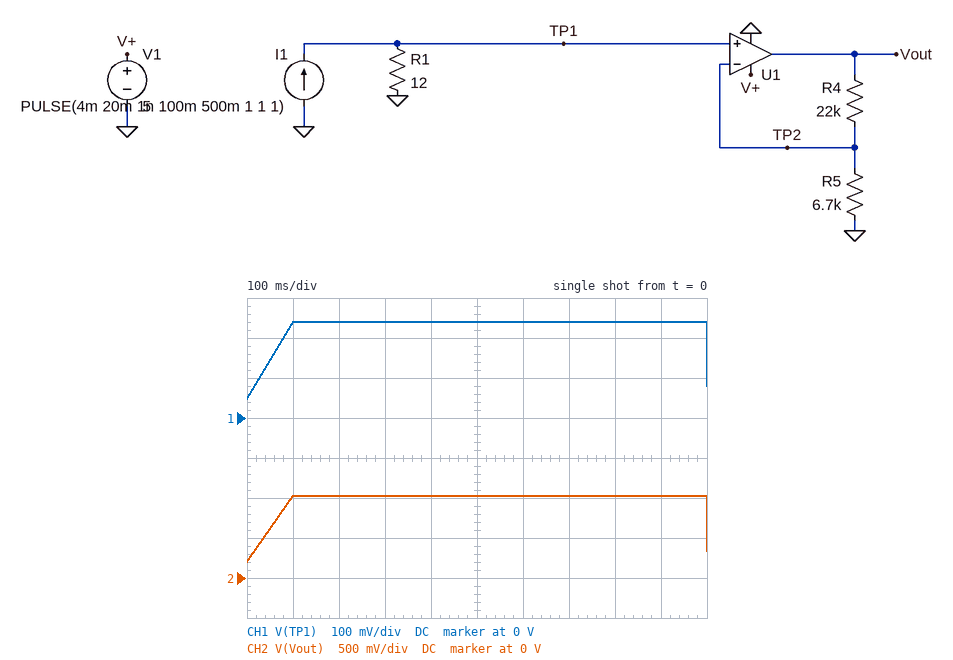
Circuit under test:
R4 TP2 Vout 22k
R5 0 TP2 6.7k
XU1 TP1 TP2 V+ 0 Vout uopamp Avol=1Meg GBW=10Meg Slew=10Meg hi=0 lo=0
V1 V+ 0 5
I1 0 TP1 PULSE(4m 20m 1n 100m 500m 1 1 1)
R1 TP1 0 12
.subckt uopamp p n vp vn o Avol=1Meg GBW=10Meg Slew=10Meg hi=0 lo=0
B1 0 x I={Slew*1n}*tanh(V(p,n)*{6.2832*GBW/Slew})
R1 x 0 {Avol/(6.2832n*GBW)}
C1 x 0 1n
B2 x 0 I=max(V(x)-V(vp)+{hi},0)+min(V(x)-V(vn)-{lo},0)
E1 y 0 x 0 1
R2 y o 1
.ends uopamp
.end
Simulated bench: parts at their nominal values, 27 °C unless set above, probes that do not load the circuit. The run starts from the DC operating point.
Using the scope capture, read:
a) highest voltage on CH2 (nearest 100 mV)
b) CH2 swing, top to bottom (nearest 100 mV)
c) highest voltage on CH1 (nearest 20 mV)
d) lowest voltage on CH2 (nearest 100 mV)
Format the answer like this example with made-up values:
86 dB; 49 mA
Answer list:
1.0 V; 800 mV; 240 mV; 200 mV
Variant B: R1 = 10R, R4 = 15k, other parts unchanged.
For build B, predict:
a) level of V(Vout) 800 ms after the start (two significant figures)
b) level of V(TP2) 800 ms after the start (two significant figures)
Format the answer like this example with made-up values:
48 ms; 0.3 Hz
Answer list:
650 mV; 200 mV
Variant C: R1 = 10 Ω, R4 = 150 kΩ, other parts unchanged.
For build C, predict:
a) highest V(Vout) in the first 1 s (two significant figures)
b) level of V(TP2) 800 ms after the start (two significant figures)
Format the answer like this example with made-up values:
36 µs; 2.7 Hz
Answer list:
4.7 V; 200 mV
